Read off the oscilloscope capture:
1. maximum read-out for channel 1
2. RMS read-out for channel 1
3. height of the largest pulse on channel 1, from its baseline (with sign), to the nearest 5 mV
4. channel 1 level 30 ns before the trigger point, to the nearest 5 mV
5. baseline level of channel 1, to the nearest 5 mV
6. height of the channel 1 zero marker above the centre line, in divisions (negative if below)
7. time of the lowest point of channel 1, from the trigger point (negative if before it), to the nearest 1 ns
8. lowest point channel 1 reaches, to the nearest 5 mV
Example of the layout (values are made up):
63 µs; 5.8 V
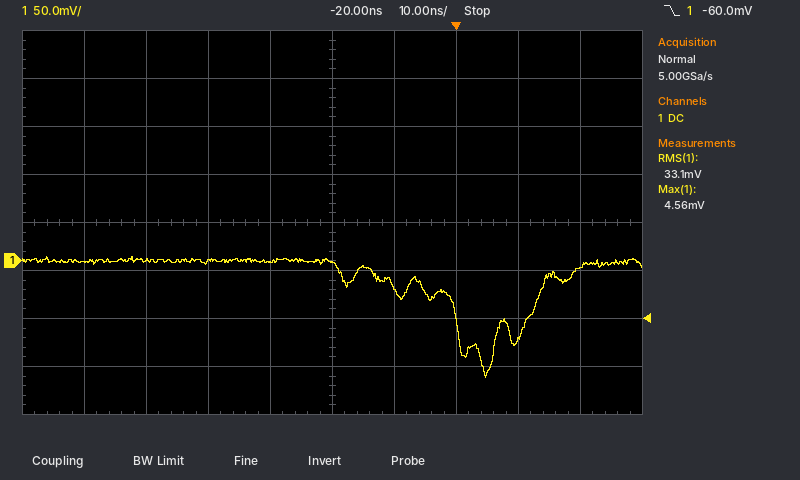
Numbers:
4.56 mV; 33.1 mV; -120 mV; 0 mV; 0 mV; -0.8 div; +5 ns; -120 mV
